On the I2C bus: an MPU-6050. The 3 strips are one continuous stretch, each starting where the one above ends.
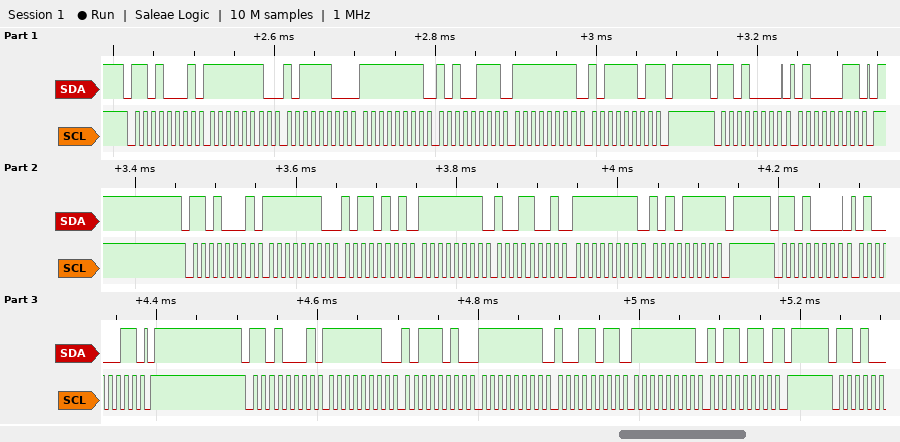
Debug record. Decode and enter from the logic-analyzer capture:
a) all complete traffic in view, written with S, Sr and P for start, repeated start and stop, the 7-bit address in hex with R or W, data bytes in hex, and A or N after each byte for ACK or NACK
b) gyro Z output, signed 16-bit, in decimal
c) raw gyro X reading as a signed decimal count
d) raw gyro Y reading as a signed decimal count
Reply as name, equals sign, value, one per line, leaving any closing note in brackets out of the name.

all complete traffic in view, written with S, Sr and P for start, repeated start and stop, the 7-bit address in hex with R or W, data bytes in hex, and A or N after each byte for ACK or NACK = S 68R A FE A BC A FF A A7 A FF A BD N P S 68W A 43 A P S 68R A FE A B5 A FF A 99 A FF A AF N P S 68W A 43 A P S 68R A FE A BA A FF A 9B A FF A B6 N P
gyro Z output, signed 16-bit, in decimal = -81
raw gyro X reading as a signed decimal count = -331
raw gyro Y reading as a signed decimal count = -103
